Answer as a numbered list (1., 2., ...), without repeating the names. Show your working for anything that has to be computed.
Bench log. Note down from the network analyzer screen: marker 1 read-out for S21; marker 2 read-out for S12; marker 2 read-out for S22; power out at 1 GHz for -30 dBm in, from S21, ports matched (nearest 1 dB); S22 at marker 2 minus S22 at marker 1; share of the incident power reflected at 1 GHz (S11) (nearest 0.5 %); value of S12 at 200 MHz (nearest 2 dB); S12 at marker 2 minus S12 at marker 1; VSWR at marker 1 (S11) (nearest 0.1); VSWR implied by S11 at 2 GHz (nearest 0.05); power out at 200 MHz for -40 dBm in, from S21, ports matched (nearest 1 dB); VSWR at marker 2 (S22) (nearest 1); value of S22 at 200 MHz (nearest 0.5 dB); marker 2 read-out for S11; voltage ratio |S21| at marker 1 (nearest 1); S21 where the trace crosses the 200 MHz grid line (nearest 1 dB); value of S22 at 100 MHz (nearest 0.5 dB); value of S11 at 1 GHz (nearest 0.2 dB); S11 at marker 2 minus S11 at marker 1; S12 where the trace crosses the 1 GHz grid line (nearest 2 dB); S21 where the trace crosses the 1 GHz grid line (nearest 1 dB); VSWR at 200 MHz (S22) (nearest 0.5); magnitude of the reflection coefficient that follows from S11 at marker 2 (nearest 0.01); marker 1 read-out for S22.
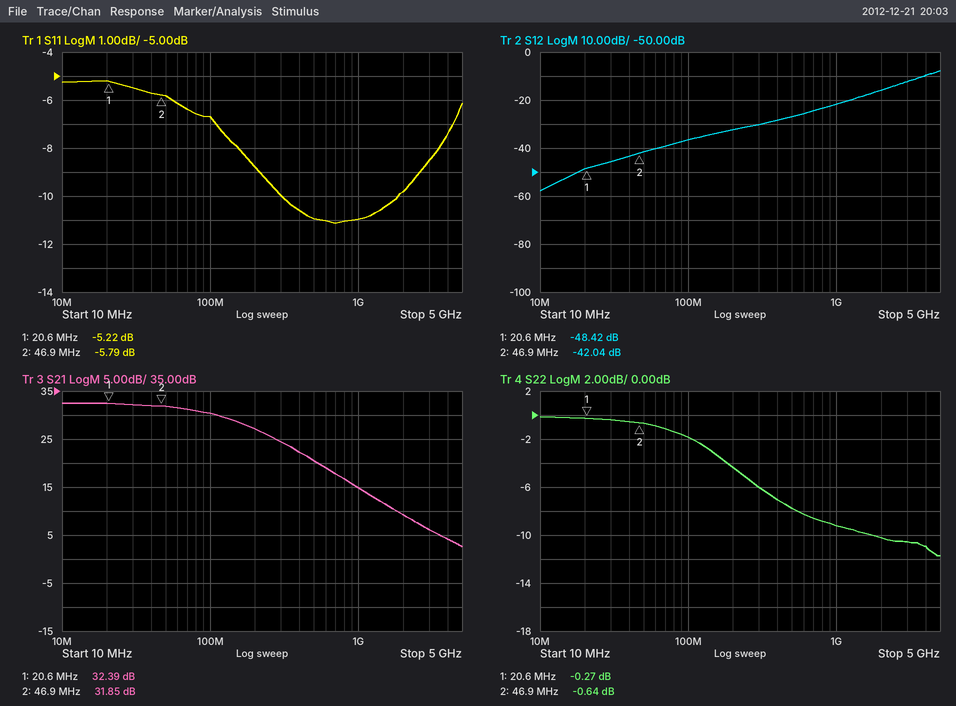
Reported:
1. 32.39 dB
2. -42.04 dB
3. -0.64 dB
4. -30 dBm + (15 dB) = -15 dBm
5. -0.64 − (-0.27) = -0.37 dB
6. 10^(-11/10) ≈ 7.94 %, so 8.0 % to the nearest 0.5 %
7. -32 dB
8. -42.04 − (-48.42) = 6.38 dB
9. (1 + 0.5483)/(1 − 0.5483) ≈ 3.4
10. |Γ| = 10^(-9.8/20) = 0.3236; VSWR = (1 + 0.3236)/(1 − 0.3236) ≈ 1.96, so 1.95 to the nearest 0.05
11. -40 dBm + (27 dB) = -13 dBm
12. (1 + 0.9290)/(1 − 0.9290) ≈ 27
13. -4.5 dB
14. -5.79 dB
15. 10^(32.39/20) ≈ 42
16. 27 dB
17. -2.0 dB
18. -11.0 dB
19. -5.79 − (-5.22) = -0.57 dB
20. -22 dB
21. 15 dB
22. |Γ| = 10^(-4.5/20) = 0.5957; VSWR = (1 + 0.5957)/(1 − 0.5957) ≈ 4.0
23. 10^(-5.79/20) ≈ 0.51
24. -0.27 dB
